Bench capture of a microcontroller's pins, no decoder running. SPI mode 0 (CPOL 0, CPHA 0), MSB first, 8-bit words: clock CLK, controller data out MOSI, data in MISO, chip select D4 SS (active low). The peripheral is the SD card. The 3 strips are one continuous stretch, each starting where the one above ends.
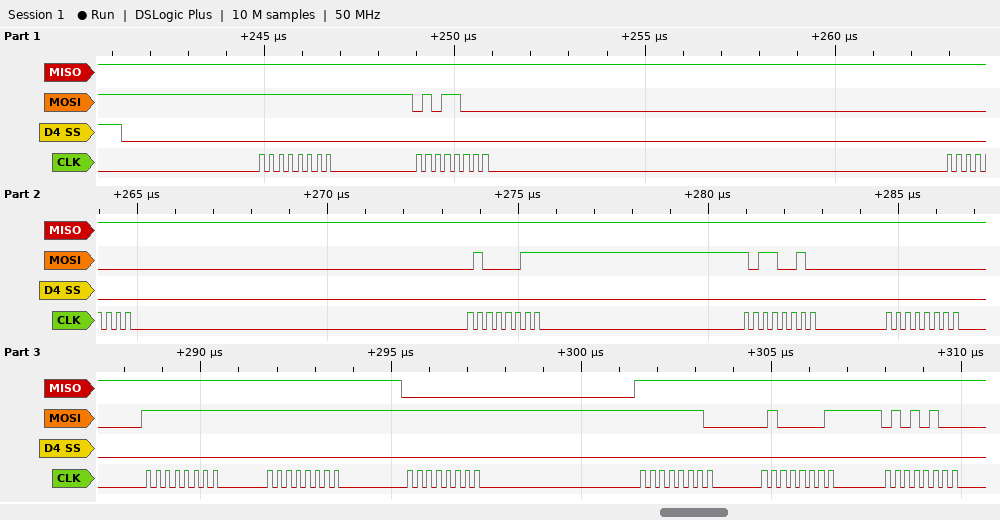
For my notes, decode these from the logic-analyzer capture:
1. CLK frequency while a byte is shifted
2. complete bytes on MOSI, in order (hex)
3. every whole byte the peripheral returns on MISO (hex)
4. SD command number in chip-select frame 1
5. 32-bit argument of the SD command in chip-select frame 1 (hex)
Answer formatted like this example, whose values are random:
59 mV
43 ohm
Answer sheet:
4 MHz
FF 58 00 43 B2 00 FF FF FF FE 41 54
FF FF FF FF FF FF FF FF 00 FF FF FF
CMD24
0x0043B200
